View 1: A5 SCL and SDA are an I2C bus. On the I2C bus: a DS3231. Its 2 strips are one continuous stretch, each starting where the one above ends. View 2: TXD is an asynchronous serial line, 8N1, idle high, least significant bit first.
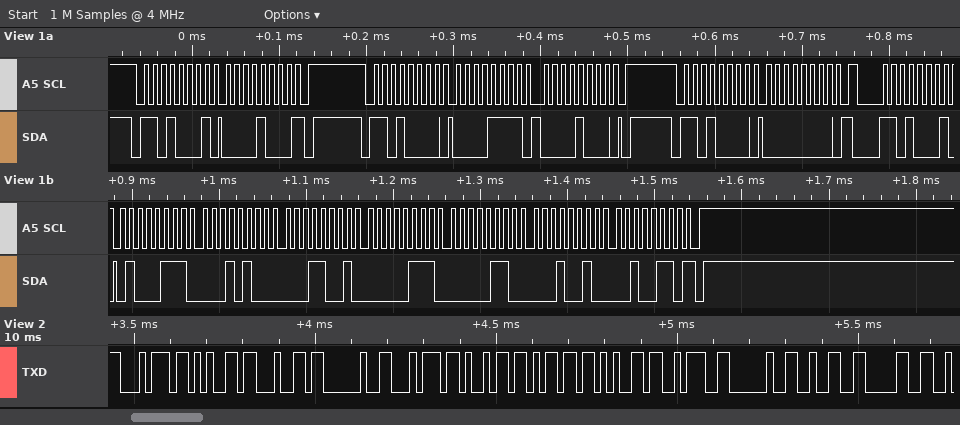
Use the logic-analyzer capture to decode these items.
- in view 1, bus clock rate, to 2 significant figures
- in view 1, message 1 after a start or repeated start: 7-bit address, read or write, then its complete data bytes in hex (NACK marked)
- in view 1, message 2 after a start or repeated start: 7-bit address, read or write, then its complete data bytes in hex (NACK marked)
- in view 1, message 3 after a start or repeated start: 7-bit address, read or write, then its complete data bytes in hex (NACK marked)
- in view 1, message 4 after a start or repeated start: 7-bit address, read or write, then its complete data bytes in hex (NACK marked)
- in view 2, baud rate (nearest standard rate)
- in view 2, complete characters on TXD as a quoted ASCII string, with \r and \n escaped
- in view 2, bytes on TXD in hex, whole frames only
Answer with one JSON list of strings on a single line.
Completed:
["100 kHz", "0x68 read: 08 NACK", "0x68 write: 0F 08", "0x68 write: 00", "0x68 read: 47 14 19 07 06 12 26 NACK", "57600 baud", "\"ted time: 20\"", "74 65 64 20 74 69 6D 65 3A 20 32 30"]
